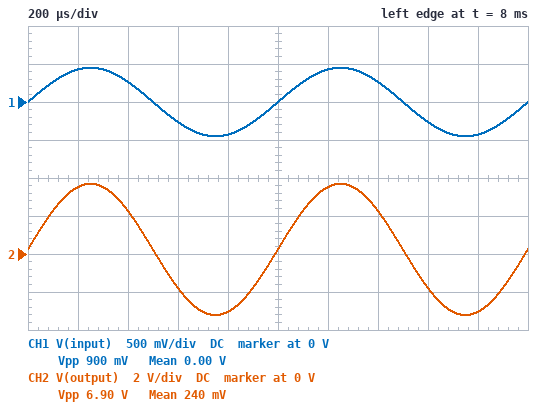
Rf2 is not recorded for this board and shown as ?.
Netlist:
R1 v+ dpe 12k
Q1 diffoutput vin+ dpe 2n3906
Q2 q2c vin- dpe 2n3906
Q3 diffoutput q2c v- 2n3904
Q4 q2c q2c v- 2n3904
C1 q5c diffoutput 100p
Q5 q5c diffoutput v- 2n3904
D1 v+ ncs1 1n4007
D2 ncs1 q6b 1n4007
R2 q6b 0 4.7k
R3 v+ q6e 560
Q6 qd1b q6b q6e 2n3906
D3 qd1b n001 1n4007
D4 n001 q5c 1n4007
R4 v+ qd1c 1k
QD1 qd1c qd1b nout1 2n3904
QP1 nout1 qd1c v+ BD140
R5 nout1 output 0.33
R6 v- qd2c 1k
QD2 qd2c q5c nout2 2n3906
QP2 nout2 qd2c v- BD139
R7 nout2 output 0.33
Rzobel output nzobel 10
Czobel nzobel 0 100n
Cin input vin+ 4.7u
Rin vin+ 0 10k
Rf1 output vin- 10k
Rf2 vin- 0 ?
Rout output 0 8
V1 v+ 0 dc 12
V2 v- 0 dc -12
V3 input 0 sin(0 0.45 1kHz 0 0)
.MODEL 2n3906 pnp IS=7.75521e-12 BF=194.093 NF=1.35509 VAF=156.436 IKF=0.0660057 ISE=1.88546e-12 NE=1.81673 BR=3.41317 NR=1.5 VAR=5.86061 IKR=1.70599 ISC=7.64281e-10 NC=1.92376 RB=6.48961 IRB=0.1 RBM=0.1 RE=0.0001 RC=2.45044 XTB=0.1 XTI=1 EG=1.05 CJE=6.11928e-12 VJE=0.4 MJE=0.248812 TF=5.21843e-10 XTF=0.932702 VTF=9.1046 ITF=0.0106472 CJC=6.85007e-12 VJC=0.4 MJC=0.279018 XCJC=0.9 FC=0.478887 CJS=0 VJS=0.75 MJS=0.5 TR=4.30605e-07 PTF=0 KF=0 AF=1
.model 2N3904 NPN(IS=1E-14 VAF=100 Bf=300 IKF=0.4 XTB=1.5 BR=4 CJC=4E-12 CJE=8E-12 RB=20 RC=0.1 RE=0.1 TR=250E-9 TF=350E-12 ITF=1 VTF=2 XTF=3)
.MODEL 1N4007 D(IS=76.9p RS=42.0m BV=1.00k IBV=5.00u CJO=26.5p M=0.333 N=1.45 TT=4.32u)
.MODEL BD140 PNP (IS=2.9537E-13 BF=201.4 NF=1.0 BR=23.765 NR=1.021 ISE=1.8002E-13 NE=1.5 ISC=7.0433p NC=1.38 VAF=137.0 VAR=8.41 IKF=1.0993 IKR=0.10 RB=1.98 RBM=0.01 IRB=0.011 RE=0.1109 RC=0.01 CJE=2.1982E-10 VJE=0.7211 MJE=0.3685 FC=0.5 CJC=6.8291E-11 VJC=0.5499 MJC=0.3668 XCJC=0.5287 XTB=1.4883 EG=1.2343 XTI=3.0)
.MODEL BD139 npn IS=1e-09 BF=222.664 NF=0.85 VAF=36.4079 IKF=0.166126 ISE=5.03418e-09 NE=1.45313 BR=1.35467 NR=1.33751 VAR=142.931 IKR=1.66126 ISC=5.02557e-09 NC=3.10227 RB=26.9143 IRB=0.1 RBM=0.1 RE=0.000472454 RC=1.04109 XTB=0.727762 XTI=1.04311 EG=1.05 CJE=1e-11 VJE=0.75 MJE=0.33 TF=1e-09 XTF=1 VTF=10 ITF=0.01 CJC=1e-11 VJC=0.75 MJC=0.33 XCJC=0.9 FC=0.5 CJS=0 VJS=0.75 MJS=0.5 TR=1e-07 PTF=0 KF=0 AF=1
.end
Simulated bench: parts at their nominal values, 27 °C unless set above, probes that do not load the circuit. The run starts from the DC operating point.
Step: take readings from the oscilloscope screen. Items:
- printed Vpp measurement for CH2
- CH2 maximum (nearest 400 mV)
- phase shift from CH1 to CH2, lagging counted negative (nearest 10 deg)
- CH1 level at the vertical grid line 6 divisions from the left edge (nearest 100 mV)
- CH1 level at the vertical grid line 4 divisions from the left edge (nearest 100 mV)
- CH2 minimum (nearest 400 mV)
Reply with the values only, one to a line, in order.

6.90 V
3.6 V
0 deg
400 mV
-400 mV
-3.2 V
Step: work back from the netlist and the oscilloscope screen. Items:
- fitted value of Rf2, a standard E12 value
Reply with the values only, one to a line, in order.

1.5 kΩ
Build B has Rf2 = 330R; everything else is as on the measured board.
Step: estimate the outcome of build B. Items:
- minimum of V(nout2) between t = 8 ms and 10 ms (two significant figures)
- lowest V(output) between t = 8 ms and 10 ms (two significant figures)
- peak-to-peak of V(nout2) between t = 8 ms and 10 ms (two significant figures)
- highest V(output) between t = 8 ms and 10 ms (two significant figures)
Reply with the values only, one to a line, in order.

-11 V
-10 V
21 V
10 V
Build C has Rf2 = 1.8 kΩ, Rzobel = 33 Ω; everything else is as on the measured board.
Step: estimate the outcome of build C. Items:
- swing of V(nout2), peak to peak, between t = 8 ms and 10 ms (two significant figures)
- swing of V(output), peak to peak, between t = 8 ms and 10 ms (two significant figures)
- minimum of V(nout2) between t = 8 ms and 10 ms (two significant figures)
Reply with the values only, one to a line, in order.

6.0 V
5.9 V
-2.9 V
